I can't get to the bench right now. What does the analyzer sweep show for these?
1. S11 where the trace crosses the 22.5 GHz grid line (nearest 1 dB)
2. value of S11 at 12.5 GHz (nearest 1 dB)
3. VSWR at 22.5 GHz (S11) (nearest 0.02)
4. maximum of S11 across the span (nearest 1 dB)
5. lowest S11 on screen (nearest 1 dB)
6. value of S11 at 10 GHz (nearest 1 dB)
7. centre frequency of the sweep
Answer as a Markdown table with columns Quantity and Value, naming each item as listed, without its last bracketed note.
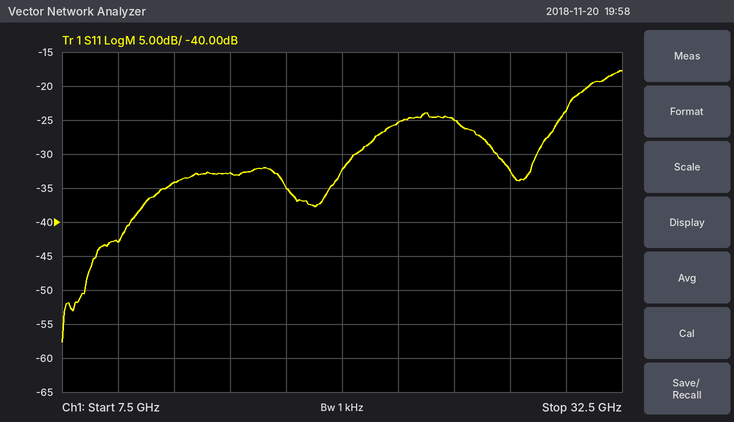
| Quantity | Value |
|---|---|
| S11 where the trace crosses the 22.5 GHz grid line | -25 dB |
| value of S11 at 12.5 GHz | -34 dB |
| VSWR at 22.5 GHz (S11) | 1.12 |
| maximum of S11 across the span | -18 dB |
| lowest S11 on screen | -58 dB |
| value of S11 at 10 GHz | -43 dB |
| centre frequency of the sweep | 20 GHz |
